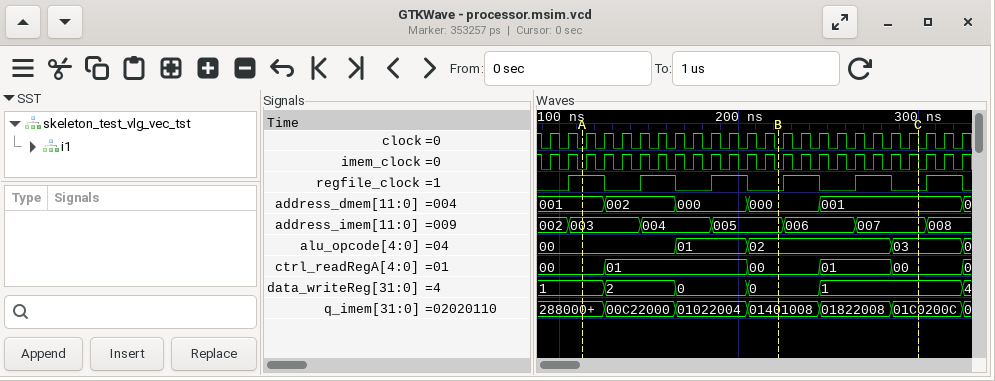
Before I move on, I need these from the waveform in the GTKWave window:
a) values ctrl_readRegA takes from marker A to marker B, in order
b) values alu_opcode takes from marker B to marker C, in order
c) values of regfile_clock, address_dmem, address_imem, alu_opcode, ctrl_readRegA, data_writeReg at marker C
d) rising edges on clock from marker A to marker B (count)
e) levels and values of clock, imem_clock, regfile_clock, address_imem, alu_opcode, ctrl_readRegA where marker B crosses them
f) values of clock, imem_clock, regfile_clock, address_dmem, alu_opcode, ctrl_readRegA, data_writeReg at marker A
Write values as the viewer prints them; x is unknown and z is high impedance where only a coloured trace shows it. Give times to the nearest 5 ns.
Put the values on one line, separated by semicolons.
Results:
00, 01, 00; 02, 03; regfile_clock=0, address_dmem=001, address_imem=007, alu_opcode=03, ctrl_readRegA=00, data_writeReg=1; 11; clock=0, imem_clock=0, regfile_clock=0, address_imem=005, alu_opcode=02, ctrl_readRegA=00; clock=0, imem_clock=0, regfile_clock=1, address_dmem=001, alu_opcode=00, ctrl_readRegA=00, data_writeReg=1
